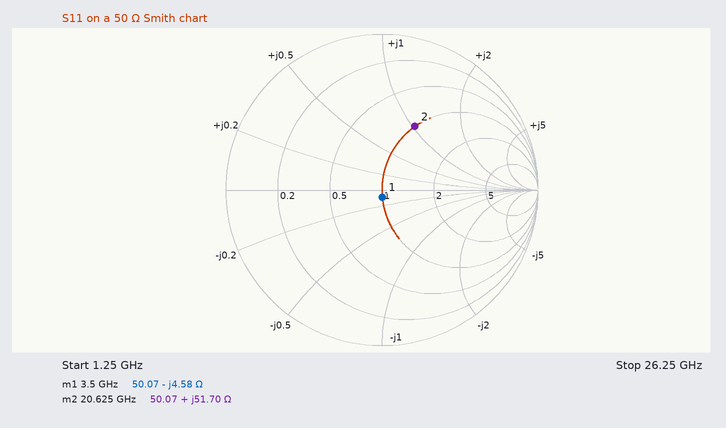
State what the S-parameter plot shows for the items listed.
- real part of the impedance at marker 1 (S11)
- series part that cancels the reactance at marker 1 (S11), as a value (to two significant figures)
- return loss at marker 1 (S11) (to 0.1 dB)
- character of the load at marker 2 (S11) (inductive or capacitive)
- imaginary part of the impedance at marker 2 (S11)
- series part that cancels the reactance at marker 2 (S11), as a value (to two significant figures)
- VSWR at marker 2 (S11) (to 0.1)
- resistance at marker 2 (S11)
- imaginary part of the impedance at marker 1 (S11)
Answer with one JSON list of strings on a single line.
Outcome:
["50.07 Ω", "210 pH", "26.8 dB", "inductive", "+51.70 Ω", "150 fF", "2.7", "50.07 Ω", "-4.58 Ω"]
